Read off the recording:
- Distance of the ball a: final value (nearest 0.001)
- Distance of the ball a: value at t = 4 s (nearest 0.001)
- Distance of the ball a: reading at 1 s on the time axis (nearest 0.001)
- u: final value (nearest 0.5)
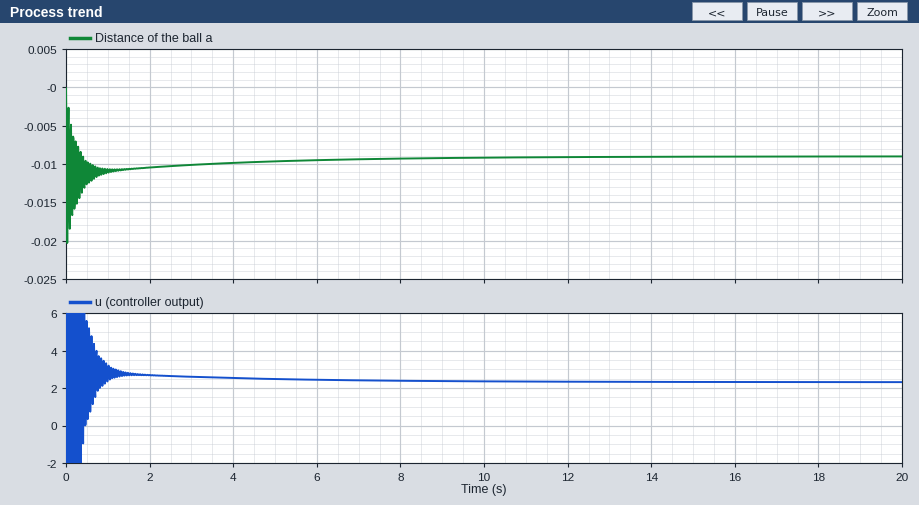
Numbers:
-0.009
-0.010
-0.011
2.5
